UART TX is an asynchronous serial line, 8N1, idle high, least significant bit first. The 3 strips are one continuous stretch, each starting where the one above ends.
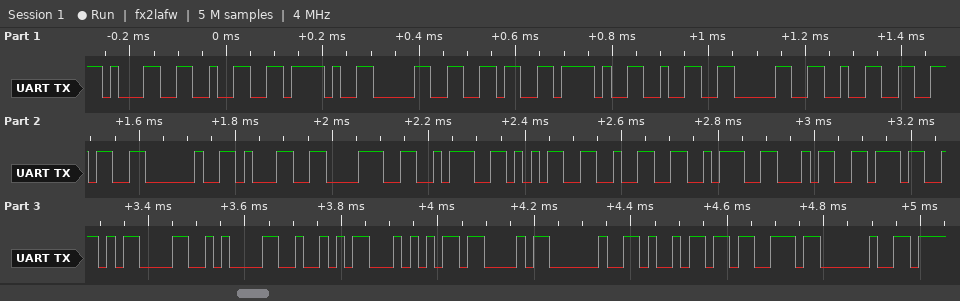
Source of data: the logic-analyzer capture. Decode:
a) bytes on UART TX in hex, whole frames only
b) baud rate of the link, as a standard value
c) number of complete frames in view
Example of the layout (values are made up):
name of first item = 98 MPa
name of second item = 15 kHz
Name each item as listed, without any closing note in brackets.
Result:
bytes on UART TX in hex, whole frames only = 31 32 2F 30 36 2F 32 30 32 36 20 31 38 3A 35 32 3A 34 37 0D 0A 52 54 43 20 69 73 20
baud rate of the link, as a standard value = 57600 baud
number of complete frames in view = 28
